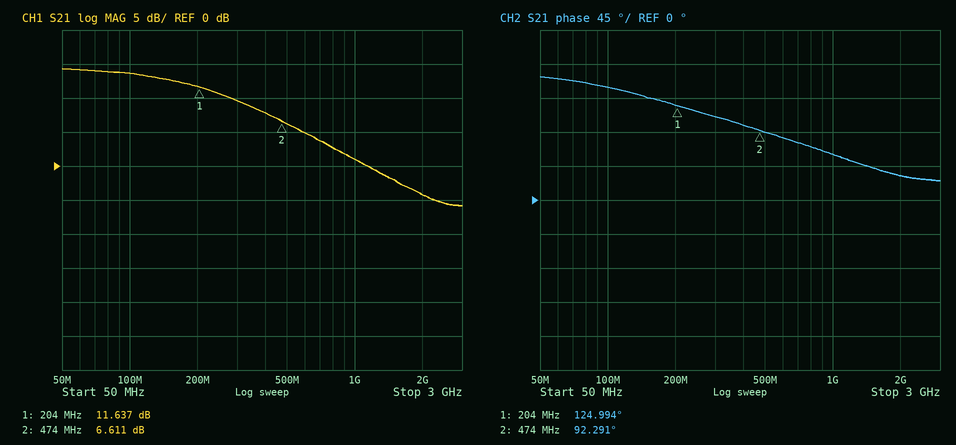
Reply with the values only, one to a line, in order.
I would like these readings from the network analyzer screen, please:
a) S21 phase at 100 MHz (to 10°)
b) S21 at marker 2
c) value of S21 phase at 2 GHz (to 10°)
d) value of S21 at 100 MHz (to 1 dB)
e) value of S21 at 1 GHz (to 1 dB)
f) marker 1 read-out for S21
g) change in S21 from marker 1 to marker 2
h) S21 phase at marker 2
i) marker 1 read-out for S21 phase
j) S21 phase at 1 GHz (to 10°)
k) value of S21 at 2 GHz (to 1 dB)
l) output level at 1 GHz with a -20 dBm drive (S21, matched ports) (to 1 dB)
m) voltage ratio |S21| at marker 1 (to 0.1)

150°
6.611 dB
30°
14 dB
1 dB
11.637 dB
-5.026 dB
92.291°
124.994°
60°
-4 dB
-19 dBm
3.8
